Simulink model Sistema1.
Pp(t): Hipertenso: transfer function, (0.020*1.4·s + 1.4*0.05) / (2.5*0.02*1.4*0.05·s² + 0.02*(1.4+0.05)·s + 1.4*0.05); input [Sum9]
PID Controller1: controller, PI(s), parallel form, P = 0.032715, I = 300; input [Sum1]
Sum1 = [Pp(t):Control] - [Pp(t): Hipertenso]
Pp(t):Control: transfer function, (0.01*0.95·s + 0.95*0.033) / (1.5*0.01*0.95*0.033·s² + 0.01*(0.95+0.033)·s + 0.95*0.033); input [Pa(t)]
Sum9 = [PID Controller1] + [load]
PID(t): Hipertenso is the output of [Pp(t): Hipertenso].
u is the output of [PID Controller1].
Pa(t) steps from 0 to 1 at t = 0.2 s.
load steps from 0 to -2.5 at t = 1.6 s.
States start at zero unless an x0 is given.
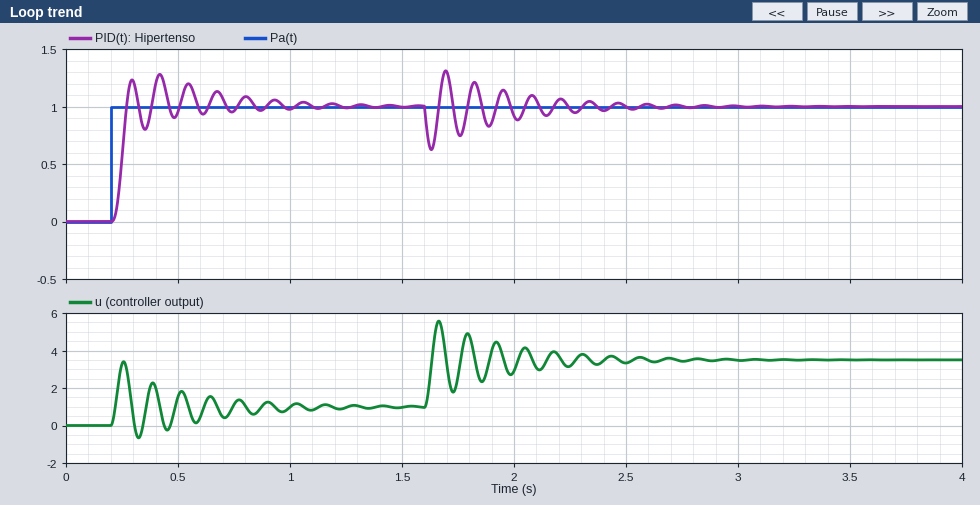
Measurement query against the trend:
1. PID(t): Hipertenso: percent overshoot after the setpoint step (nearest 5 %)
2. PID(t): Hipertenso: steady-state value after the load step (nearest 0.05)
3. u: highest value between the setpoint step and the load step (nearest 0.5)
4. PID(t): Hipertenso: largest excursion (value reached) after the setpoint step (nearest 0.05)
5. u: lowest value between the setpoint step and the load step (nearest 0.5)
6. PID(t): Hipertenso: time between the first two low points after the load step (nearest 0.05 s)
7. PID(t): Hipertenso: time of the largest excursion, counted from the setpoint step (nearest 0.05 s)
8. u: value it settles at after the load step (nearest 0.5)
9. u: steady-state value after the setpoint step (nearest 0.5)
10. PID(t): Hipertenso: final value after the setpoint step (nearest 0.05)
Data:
30 %
1.00
3.5
1.30
-0.5
0.15 s
0.20 s
3.5
1.0
1.00
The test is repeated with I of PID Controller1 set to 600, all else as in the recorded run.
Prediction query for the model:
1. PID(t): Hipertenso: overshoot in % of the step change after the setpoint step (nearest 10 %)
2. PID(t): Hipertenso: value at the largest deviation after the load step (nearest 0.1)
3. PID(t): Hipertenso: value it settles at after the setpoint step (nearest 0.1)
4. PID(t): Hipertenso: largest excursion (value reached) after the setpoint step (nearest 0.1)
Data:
20 %
0.7
1.0
1.2
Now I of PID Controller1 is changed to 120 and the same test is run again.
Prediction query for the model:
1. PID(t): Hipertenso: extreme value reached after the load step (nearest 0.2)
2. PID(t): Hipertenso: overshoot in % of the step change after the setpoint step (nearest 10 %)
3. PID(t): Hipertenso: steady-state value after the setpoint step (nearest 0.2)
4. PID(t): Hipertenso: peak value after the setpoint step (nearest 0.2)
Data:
0.4
40 %
1.0
1.4
